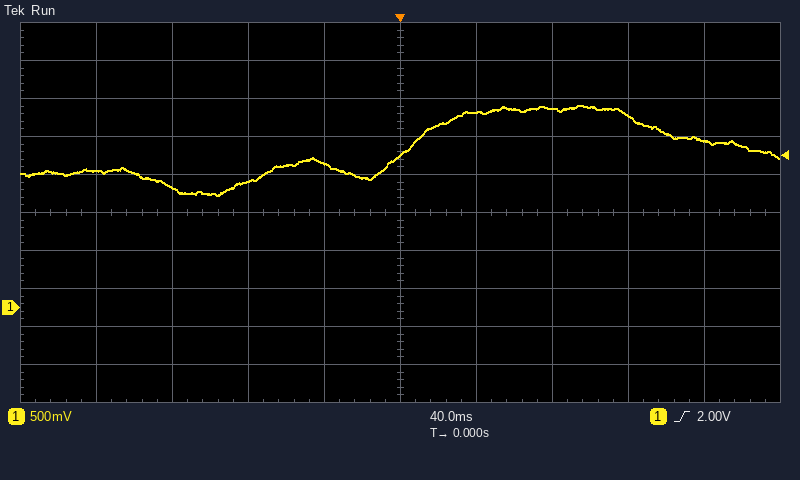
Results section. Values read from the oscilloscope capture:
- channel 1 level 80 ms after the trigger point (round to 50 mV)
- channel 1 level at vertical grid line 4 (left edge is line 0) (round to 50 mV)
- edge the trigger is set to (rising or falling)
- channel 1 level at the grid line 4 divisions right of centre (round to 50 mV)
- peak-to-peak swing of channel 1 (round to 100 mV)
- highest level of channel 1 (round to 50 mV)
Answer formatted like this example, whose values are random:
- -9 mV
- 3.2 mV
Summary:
- 2.60 V
- 1.90 V
- rising
- 2.20 V
- 1.20 V
- 2.65 V
